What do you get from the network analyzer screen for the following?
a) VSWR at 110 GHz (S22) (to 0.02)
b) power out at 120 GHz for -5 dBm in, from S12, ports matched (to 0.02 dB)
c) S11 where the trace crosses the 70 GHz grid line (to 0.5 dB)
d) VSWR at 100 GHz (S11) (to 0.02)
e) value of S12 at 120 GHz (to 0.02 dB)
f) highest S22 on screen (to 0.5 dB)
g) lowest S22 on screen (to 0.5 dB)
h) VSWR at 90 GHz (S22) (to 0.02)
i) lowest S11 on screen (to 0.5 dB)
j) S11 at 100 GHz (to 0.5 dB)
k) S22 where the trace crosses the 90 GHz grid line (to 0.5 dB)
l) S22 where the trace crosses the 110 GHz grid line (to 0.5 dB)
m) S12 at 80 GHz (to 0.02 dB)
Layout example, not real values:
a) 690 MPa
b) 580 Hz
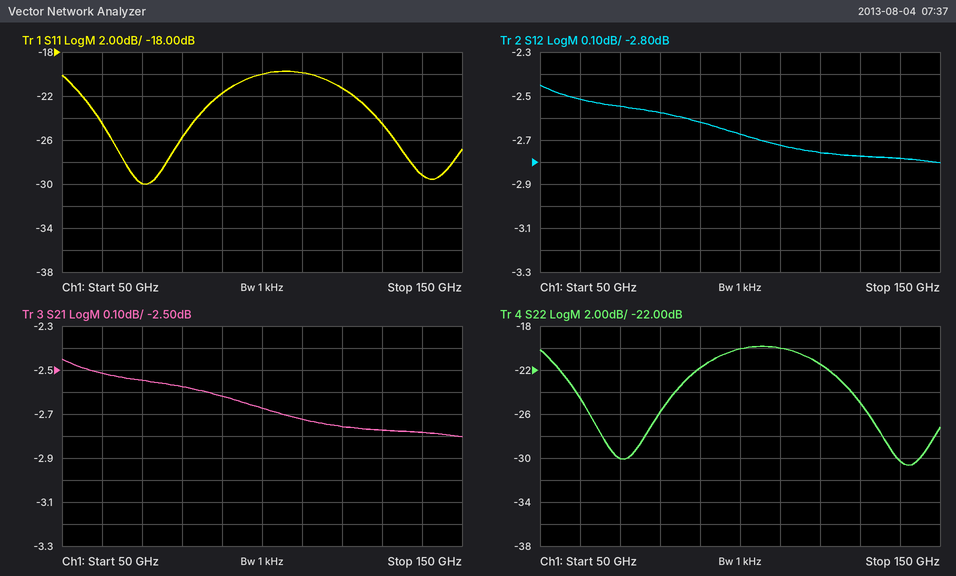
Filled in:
a) 1.22
b) -7.76 dBm
c) -30.0 dB
d) 1.22
e) -2.76 dB
f) -20.0 dB
g) -30.5 dB
h) 1.18
i) -30.0 dB
j) -20.0 dB
k) -22.0 dB
l) -20.0 dB
m) -2.58 dB
